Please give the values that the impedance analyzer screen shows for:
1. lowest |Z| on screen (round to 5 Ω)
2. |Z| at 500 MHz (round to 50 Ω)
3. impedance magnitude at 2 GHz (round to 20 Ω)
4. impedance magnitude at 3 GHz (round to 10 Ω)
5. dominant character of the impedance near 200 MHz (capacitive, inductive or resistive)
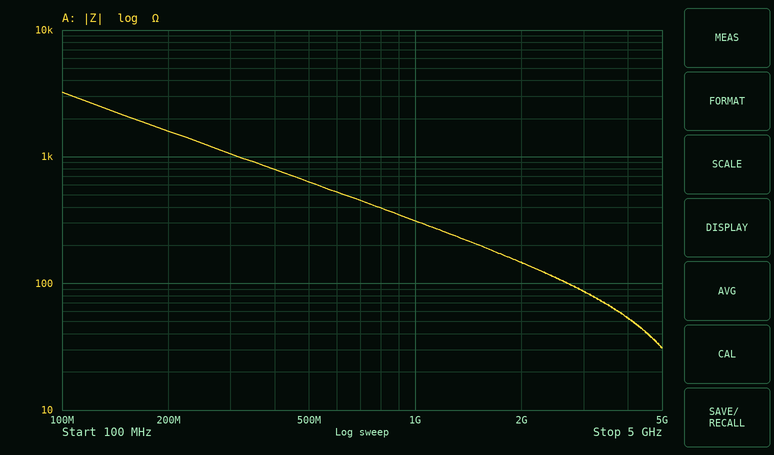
30 Ω
650 Ω
140 Ω
90 Ω
capacitive
